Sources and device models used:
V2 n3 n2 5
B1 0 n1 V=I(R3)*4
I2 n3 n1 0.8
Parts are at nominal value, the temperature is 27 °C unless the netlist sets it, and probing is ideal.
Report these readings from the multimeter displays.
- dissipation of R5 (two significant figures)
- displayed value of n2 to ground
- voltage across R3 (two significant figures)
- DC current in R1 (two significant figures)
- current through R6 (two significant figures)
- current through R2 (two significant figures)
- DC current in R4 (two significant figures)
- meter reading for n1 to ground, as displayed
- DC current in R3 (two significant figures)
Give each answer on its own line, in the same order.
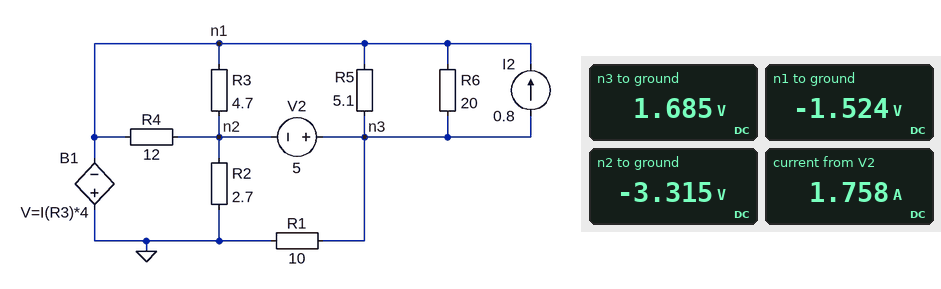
2.0 W
-3.315 V
1.8 V
170 mA
160 mA
1.2 A
150 mA
-1.524 V
380 mA
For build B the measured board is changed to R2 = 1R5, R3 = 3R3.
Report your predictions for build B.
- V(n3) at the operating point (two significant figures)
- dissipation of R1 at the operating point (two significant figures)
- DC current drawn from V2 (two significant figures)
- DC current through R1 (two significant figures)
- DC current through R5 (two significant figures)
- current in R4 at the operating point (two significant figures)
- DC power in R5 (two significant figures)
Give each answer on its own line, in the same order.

2.6 V
670 mW
2.0 A
260 mA
770 mA
91 mA
3.0 W
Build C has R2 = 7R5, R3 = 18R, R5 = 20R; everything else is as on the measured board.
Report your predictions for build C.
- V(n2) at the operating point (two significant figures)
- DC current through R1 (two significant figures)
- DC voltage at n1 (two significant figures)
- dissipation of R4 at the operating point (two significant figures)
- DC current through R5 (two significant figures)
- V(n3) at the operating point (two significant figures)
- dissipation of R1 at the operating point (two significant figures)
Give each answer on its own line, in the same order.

-4.2 V
80 mA
-760 mV
980 mW
78 mA
800 mV
64 mW
